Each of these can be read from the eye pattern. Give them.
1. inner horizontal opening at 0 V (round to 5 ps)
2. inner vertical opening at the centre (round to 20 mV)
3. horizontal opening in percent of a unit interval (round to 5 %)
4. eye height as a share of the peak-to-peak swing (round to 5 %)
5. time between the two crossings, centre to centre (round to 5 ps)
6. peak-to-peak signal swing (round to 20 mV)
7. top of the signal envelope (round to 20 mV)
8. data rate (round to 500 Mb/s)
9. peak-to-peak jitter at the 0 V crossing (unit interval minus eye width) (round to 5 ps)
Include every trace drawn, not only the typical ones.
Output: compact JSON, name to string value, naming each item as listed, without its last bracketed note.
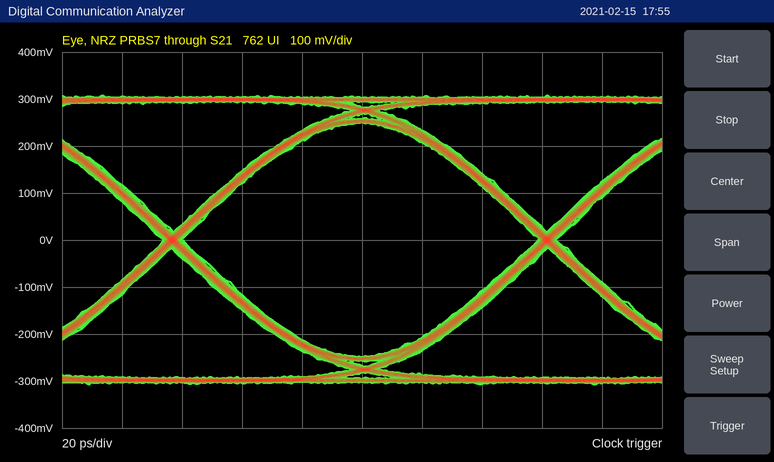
{"inner horizontal opening at 0 V": "120 ps", "inner vertical opening at the centre": "500 mV", "horizontal opening in percent of a unit interval": "95 %", "eye height as a share of the peak-to-peak swing": "80 %", "time between the two crossings, centre to centre": "125 ps", "peak-to-peak signal swing": "620 mV", "top of the signal envelope": "300 mV", "data rate": "8.0 Gb/s", "peak-to-peak jitter at the 0 V crossing (unit interval minus eye width)": "5 ps"}
